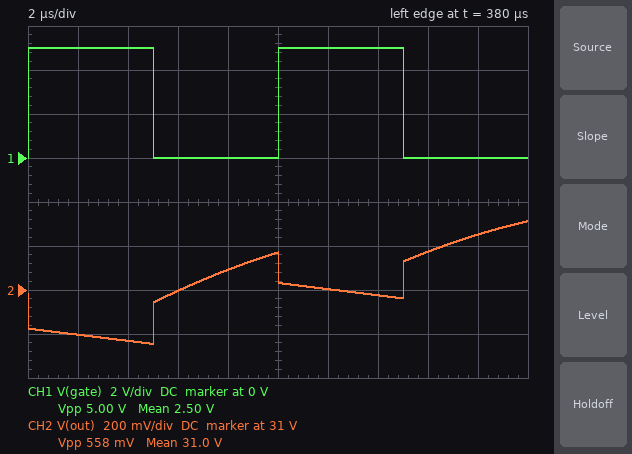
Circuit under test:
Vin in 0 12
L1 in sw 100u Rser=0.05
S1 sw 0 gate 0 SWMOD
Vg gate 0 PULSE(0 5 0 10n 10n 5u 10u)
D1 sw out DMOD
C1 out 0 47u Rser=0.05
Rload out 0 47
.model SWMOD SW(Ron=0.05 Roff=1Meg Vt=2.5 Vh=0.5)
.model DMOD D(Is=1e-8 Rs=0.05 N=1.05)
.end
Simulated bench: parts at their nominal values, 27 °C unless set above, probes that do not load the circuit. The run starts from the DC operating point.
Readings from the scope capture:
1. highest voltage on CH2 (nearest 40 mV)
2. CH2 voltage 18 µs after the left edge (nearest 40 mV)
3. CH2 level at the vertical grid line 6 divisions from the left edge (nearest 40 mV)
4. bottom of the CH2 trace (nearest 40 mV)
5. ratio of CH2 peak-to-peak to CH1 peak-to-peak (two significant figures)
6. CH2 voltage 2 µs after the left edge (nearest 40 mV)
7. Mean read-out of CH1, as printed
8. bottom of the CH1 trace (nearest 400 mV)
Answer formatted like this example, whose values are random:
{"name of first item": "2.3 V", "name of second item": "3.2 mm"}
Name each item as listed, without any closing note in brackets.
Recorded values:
{"highest voltage on CH2": "31.32 V", "CH2 voltage 18 µs after the left edge": "31.24 V", "CH2 level at the vertical grid line 6 divisions from the left edge": "31.00 V", "bottom of the CH2 trace": "30.76 V", "ratio of CH2 peak-to-peak to CH1 peak-to-peak": "0.11", "CH2 voltage 2 µs after the left edge": "30.80 V", "Mean read-out of CH1, as printed": "2.50 V", "bottom of the CH1 trace": "0 V"}
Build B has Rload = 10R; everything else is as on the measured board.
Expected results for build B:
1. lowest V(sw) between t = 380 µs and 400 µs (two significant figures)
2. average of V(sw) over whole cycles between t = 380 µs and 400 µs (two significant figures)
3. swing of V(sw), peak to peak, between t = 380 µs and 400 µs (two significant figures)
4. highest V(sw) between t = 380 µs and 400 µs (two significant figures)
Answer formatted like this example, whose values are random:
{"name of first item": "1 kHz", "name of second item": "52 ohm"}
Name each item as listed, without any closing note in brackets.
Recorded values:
{"lowest V(sw) between t = 380 µs and 400 µs": "350 mV", "average of V(sw) over whole cycles between t = 380 µs and 400 µs": "14 V", "swing of V(sw), peak to peak, between t = 380 µs and 400 µs": "28 V", "highest V(sw) between t = 380 µs and 400 µs": "29 V"}
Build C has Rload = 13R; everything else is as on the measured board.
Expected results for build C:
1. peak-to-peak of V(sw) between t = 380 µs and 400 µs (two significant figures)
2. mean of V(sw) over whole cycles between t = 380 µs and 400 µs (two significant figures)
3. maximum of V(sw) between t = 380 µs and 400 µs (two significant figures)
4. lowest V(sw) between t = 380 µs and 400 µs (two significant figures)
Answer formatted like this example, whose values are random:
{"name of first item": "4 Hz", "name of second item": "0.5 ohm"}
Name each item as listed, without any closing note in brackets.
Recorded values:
{"peak-to-peak of V(sw) between t = 380 µs and 400 µs": "29 V", "mean of V(sw) over whole cycles between t = 380 µs and 400 µs": "15 V", "maximum of V(sw) between t = 380 µs and 400 µs": "30 V", "lowest V(sw) between t = 380 µs and 400 µs": "290 mV"}
